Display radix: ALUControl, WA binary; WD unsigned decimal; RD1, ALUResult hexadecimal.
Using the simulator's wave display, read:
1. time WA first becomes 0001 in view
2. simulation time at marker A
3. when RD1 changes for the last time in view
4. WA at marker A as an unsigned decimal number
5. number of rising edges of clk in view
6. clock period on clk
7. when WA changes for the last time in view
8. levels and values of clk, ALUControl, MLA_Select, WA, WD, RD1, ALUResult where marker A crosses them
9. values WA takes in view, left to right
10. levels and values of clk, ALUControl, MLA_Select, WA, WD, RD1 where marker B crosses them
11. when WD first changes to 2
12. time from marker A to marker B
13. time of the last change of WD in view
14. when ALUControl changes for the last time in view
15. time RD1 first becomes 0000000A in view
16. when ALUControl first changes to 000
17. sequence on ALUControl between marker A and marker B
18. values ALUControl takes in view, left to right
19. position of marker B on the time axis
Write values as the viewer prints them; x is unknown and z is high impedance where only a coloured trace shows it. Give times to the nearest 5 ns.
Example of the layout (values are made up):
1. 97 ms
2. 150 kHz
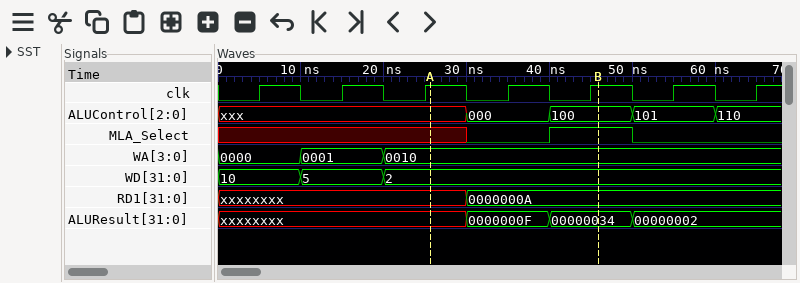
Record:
1. 10 ns
2. 25 ns
3. 30 ns
4. 2
5. 7
6. 10 ns
7. 20 ns
8. clk=1, ALUControl=xxx, MLA_Select=x, WA=0010, WD=2, RD1=xxxxxxxx, ALUResult=xxxxxxxx
9. 0000, 0001, 0010
10. clk=1, ALUControl=100, MLA_Select=1, WA=0010, WD=2, RD1=0000000A
11. 20 ns
12. 20 ns
13. 20 ns
14. 60 ns
15. 30 ns
16. 30 ns
17. xxx, 000, 100
18. xxx, 000, 100, 101, 110
19. 45 ns
